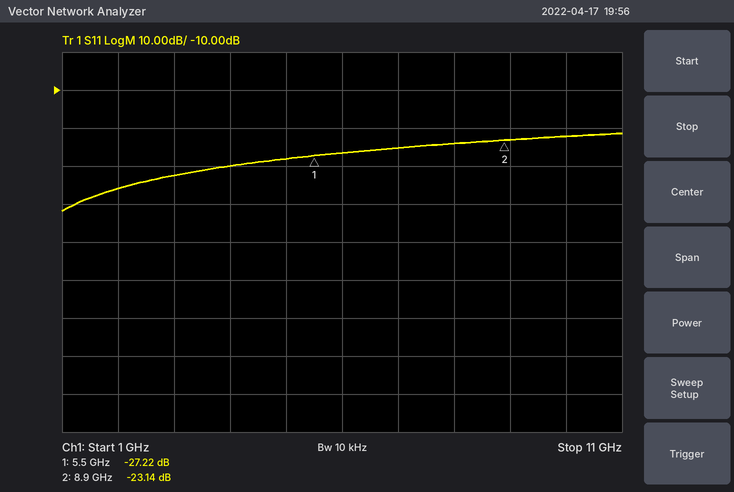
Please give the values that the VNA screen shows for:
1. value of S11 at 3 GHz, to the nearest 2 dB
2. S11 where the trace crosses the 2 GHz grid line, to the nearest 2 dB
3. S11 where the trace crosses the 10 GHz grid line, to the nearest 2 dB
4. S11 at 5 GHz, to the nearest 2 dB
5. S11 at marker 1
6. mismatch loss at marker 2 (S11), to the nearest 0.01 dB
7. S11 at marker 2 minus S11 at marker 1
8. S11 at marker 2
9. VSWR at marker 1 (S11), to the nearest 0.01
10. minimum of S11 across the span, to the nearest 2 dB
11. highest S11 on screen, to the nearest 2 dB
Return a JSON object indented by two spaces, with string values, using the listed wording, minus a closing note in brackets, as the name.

{
  "value of S11 at 3 GHz, to the nearest 2 dB": "-32 dB",
  "S11 where the trace crosses the 2 GHz grid line, to the nearest 2 dB": "-36 dB",
  "S11 where the trace crosses the 10 GHz grid line, to the nearest 2 dB": "-22 dB",
  "S11 at 5 GHz, to the nearest 2 dB": "-28 dB",
  "S11 at marker 1": "-27.22 dB",
  "mismatch loss at marker 2 (S11), to the nearest 0.01 dB": "0.02 dB",
  "S11 at marker 2 minus S11 at marker 1": "4.08 dB",
  "S11 at marker 2": "-23.14 dB",
  "VSWR at marker 1 (S11), to the nearest 0.01": "1.09",
  "minimum of S11 across the span, to the nearest 2 dB": "-42 dB",
  "highest S11 on screen, to the nearest 2 dB": "-22 dB"
}
